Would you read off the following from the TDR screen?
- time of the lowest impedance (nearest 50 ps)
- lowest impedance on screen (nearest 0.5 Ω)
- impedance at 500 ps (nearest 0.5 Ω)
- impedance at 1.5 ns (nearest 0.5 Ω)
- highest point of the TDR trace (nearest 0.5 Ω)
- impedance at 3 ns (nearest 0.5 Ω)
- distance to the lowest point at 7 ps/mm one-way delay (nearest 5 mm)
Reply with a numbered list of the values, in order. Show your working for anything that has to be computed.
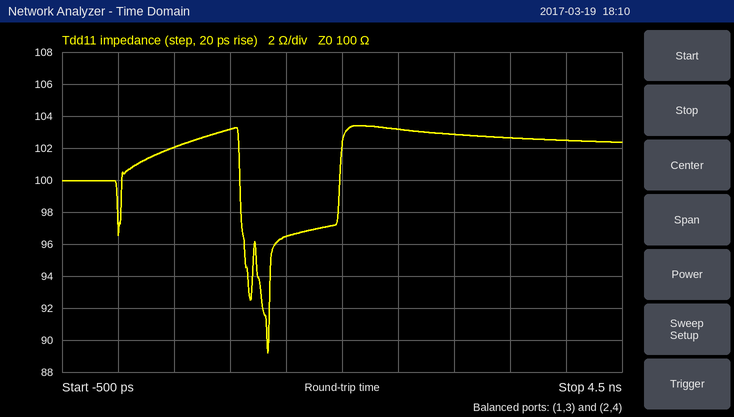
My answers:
1. 1.35 ns
2. 89.0 Ω
3. 102.0 Ω
4. 96.5 Ω
5. 103.5 Ω
6. 103.0 Ω
7. 1.35 ns / 2 / 7 ps/mm ≈ 96.4 mm, so 95 mm to the nearest 5 mm
